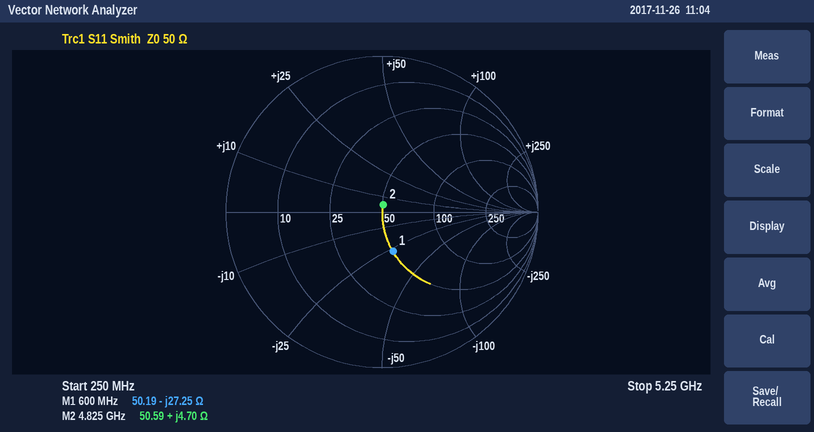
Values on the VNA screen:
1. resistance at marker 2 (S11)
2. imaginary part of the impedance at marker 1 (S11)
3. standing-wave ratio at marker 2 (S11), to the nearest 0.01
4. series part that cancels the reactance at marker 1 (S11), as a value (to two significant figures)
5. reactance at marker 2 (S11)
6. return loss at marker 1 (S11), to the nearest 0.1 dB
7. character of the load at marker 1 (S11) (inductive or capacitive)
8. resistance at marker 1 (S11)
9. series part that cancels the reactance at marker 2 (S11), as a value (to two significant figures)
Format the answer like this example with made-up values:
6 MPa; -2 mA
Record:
50.59 Ω; -27.25 Ω; 1.10; 7.2 nH; +4.70 Ω; 11.6 dB; capacitive; 50.19 Ω; 7.0 pF
